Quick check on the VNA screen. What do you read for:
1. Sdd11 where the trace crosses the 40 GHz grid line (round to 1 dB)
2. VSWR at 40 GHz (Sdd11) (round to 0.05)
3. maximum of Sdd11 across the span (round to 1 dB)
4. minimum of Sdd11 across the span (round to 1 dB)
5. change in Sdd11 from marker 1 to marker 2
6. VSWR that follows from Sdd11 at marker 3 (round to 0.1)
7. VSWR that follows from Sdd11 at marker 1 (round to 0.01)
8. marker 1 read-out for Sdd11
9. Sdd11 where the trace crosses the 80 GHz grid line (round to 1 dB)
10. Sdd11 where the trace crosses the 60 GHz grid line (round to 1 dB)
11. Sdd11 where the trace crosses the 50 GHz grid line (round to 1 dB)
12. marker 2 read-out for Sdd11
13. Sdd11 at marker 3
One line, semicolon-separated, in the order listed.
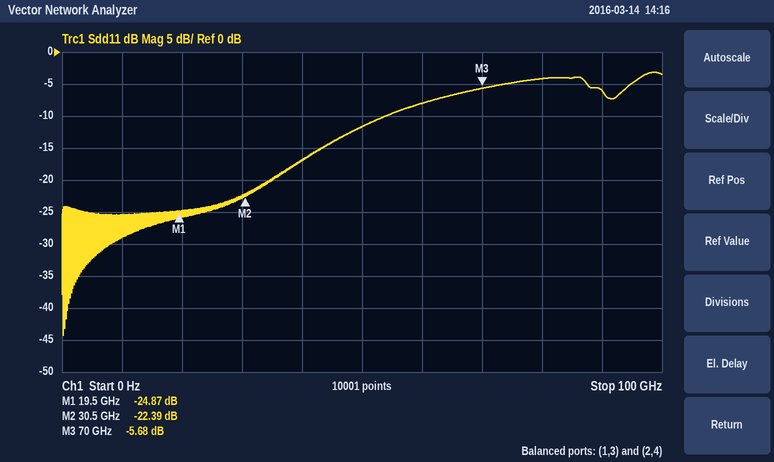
-17 dB; 1.35; -3 dB; -44 dB; 2.48 dB; 3.2; 1.12; -24.87 dB; -4 dB; -8 dB; -12 dB; -22.39 dB; -5.68 dB
